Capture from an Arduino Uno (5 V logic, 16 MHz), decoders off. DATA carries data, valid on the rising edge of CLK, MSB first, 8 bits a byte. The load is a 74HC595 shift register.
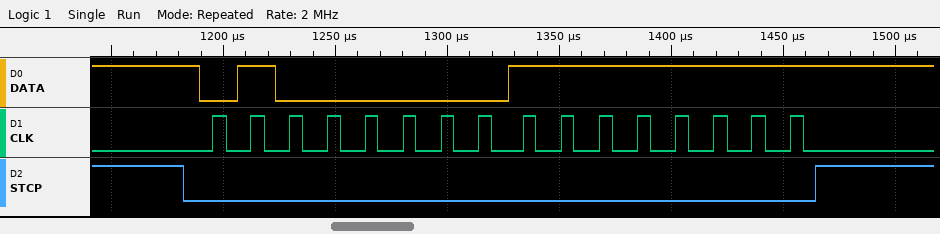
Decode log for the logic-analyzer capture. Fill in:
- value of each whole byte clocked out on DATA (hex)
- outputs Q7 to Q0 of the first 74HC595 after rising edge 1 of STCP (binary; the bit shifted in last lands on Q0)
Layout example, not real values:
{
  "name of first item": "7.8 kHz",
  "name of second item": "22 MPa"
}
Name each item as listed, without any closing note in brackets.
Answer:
{
  "value of each whole byte clocked out on DATA": "0x40 0xFF",
  "outputs Q7 to Q0 of the first 74HC595 after rising edge 1 of STCP": "11111111"
}
